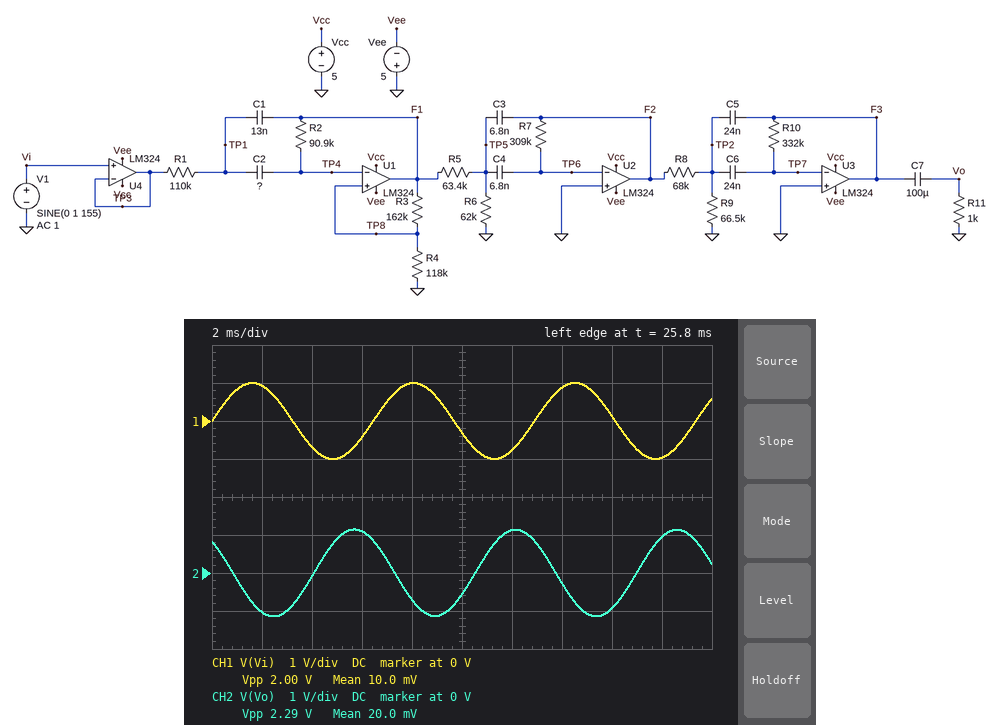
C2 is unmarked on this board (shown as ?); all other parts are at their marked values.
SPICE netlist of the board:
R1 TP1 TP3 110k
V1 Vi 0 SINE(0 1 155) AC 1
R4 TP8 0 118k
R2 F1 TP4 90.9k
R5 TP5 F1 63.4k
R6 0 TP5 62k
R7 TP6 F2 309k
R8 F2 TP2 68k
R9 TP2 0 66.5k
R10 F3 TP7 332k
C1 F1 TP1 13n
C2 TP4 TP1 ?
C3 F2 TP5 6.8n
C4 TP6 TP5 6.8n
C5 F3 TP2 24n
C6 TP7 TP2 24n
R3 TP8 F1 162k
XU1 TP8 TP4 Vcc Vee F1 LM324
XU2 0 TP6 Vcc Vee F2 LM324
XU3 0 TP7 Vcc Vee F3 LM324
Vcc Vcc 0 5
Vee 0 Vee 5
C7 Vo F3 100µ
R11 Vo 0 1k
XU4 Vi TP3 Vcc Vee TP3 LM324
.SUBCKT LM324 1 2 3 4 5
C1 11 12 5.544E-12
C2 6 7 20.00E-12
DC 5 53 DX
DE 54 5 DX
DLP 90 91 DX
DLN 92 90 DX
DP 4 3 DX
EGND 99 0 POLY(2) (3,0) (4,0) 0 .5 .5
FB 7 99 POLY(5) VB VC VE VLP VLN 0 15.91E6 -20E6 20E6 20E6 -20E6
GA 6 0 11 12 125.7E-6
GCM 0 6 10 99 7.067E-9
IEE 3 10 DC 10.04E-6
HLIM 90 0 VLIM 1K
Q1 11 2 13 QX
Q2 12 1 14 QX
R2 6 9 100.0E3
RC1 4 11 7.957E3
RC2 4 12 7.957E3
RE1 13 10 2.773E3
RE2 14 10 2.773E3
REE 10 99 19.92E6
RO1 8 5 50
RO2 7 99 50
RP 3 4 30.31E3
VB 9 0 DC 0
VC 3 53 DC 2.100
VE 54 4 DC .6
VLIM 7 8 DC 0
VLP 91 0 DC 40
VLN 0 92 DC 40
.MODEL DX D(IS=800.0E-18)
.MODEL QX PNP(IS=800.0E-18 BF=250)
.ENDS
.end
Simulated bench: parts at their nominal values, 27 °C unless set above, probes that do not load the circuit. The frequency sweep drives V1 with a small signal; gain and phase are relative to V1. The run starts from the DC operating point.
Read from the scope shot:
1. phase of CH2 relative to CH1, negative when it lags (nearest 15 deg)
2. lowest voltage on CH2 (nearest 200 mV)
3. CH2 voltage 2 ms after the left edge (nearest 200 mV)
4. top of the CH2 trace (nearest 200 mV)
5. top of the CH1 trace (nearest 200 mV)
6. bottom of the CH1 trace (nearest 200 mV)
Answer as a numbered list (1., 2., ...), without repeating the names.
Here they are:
1. 135 deg
2. -1.2 V
3. -1.0 V
4. 1.2 V
5. 1.0 V
6. -1.0 V
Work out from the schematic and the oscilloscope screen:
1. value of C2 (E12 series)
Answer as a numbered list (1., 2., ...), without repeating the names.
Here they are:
1. 18 nF
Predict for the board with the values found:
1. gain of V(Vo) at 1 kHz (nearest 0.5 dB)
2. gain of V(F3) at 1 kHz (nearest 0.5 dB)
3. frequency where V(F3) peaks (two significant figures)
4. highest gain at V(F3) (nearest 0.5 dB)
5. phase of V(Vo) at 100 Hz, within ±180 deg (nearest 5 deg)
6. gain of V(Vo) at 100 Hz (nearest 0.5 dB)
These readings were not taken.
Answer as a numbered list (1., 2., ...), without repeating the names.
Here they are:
1. -43.0 dB
2. -43.0 dB
3. 82 Hz
4. 2.5 dB
5. -160 deg
6. 2.0 dB
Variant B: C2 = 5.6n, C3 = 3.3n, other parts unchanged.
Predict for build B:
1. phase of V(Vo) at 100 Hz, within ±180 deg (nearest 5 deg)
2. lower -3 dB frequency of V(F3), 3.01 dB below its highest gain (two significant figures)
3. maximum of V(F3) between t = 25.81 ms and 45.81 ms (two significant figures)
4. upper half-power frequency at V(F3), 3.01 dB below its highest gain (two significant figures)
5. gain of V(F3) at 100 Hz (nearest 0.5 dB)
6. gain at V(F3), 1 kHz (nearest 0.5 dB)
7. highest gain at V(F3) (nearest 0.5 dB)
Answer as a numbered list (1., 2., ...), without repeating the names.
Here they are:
1. -125 deg
2. 66 Hz
3. 440 mV
4. 370 Hz
5. -8.0 dB
6. -36.5 dB
7. -6.0 dB
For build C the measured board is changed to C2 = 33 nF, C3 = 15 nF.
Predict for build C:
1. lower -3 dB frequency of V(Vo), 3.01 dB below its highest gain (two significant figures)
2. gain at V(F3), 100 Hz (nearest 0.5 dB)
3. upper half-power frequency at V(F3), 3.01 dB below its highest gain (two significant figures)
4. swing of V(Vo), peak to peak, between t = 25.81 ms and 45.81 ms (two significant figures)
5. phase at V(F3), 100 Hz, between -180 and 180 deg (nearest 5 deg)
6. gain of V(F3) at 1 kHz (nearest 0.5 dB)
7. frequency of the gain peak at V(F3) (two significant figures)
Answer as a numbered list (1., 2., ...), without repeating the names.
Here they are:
1. 57 Hz
2. 6.0 dB
3. 140 Hz
4. 2.7 V
5. 155 deg
6. -50.0 dB
7. 75 Hz
